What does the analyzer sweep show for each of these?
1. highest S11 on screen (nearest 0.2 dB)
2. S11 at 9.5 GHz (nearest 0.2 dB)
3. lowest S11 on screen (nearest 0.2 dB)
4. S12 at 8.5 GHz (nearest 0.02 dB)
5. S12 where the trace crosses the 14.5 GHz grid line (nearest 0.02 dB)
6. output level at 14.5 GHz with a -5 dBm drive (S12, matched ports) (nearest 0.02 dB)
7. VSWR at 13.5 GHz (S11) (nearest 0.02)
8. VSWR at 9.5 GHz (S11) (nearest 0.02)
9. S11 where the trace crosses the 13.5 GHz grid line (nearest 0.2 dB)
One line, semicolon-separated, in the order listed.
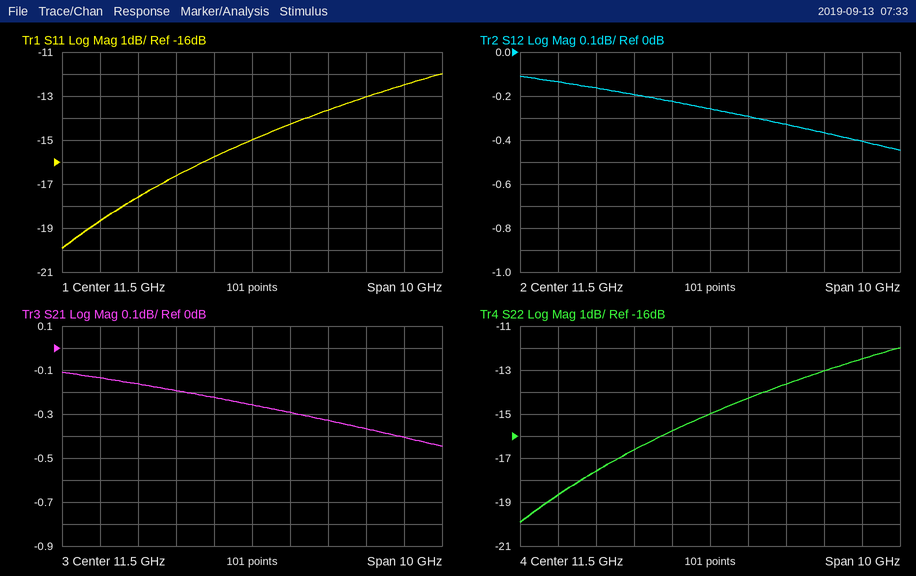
-12.0 dB; -16.6 dB; -20.0 dB; -0.16 dB; -0.36 dB; -5.36 dBm; 1.52; 1.34; -13.6 dB
